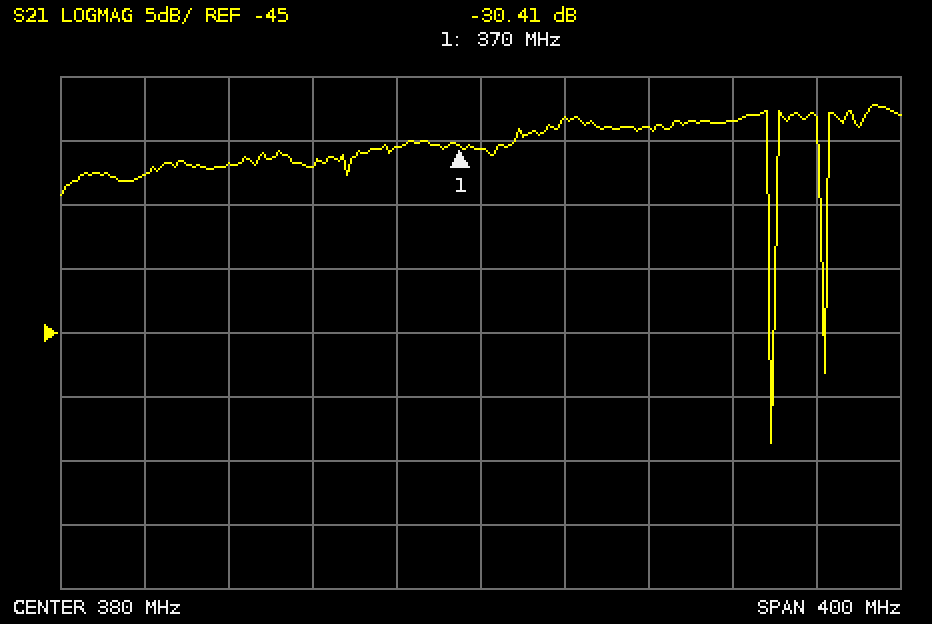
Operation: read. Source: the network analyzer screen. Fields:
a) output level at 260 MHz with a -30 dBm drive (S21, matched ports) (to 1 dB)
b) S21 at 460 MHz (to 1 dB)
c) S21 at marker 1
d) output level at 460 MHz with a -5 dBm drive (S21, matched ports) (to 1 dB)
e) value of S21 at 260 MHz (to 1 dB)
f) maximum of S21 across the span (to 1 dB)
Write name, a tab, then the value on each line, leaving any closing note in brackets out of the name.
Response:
output level at 260 MHz with a -30 dBm drive (S21, matched ports)	-62 dBm
S21 at 460 MHz	-29 dB
S21 at marker 1	-30.41 dB
output level at 460 MHz with a -5 dBm drive (S21, matched ports)	-34 dBm
value of S21 at 260 MHz	-32 dB
maximum of S21 across the span	-27 dB
